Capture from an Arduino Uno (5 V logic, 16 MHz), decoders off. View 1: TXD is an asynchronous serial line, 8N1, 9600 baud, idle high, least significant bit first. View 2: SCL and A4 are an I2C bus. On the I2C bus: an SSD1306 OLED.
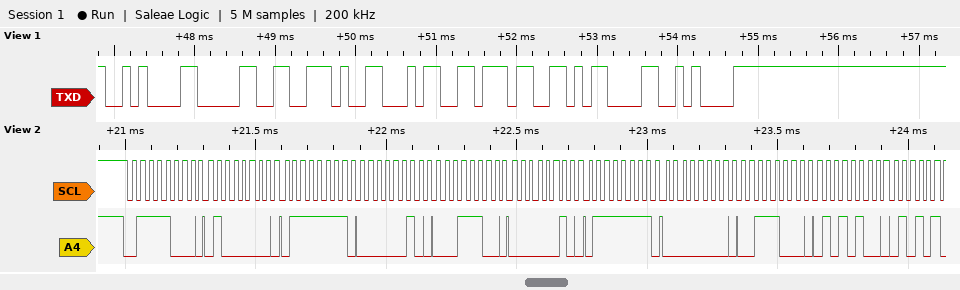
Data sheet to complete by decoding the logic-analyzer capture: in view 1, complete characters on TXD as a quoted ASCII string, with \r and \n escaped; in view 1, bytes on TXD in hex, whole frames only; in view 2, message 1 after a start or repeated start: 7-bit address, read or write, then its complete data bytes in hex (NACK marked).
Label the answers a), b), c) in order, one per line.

a) "\n0.47\r\n"
b) 0x0A 0x30 0x2E 0x34 0x37 0x0D 0x0A
c) 0x3C write: 40 7F 02 1C 02 7F 00 38 54
